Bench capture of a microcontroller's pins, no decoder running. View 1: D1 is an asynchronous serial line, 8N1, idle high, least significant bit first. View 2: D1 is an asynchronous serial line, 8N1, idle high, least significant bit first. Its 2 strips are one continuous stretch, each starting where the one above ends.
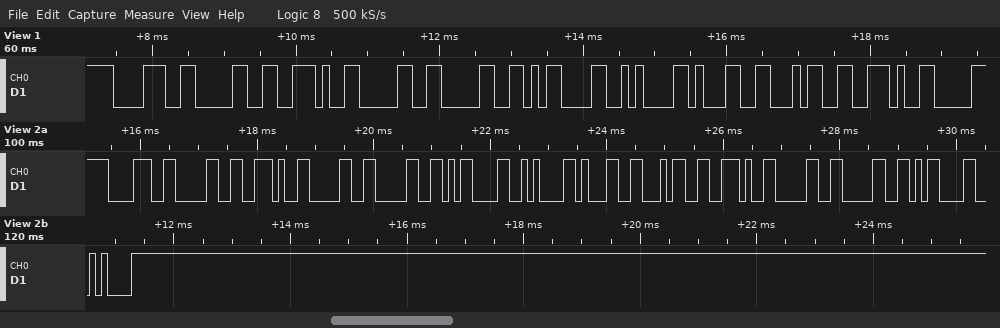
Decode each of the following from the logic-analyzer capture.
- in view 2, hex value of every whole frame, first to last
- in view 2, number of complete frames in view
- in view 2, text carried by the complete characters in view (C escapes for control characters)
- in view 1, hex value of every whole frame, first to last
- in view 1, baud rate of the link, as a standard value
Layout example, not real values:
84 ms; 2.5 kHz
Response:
38 30 2E 30 30 0D 0A 31 34 2E 30 30 0D 0A; 14; "80.00\r\n14.00\r\n"; 38 30 2E 30 30 0D 0A 31 34 2E; 9600 baud
